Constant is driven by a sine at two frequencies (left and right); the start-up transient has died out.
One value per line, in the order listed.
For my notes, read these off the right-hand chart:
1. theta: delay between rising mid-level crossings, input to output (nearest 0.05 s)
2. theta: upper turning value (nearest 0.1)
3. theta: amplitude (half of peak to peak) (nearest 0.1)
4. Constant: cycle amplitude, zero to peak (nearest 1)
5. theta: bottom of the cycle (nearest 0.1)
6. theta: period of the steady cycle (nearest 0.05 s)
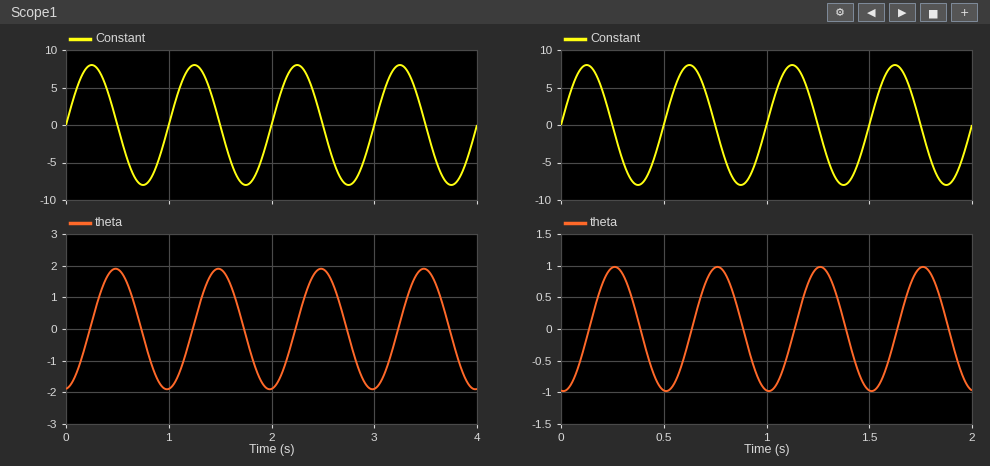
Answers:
0.15 s
1.0
1.0
8
-1.0
0.50 s
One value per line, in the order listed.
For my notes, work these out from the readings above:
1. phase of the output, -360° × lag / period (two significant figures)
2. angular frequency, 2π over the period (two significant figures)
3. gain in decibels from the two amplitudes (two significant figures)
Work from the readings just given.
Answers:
-110°
13 rad/s
-18 dB
